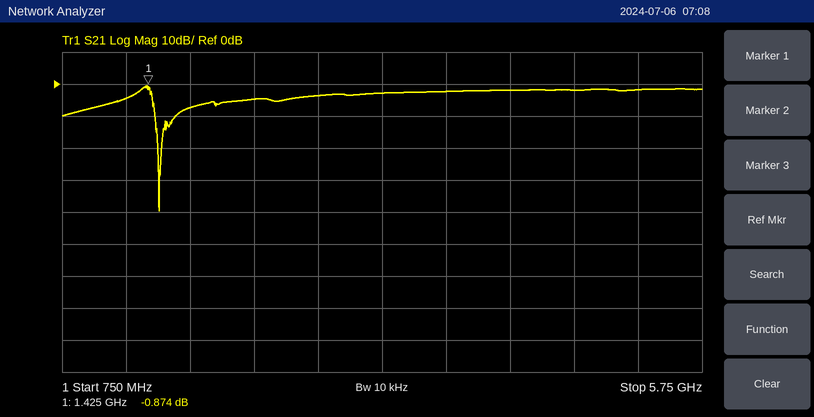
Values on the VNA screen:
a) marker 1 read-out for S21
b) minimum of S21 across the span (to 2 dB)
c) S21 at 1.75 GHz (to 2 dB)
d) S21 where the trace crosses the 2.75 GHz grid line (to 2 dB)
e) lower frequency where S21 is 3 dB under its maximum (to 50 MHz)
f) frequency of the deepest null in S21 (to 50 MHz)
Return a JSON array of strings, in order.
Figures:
["-0.874 dB", "-40 dB", "-8 dB", "-4 dB", "1.30 GHz", "1.50 GHz"]
